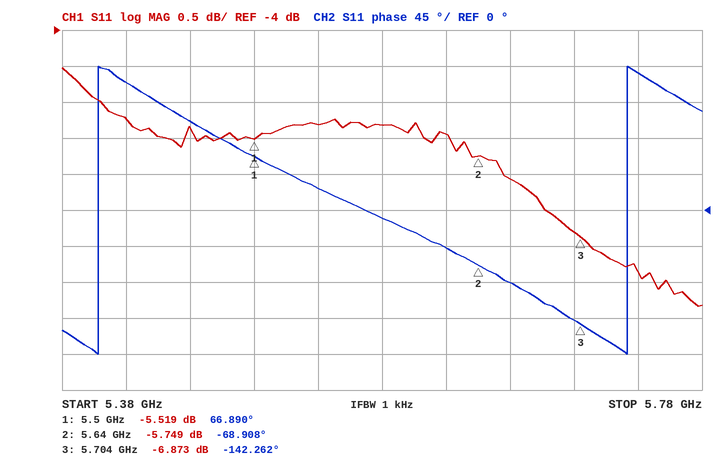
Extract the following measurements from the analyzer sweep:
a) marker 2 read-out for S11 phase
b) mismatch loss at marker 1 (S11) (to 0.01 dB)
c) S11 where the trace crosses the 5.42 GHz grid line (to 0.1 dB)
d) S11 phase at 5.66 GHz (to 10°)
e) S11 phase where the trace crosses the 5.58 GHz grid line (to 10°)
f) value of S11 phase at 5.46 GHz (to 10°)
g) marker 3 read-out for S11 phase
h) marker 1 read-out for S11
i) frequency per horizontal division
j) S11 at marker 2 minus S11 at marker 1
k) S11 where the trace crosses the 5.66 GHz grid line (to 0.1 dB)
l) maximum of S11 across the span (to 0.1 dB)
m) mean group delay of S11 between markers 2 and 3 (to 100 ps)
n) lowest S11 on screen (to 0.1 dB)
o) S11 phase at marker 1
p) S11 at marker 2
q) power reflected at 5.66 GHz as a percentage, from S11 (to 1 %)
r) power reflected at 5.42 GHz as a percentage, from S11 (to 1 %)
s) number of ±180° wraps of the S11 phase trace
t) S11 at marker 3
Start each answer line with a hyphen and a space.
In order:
- -68.908°
- 1.43 dB
- -5.2 dB
- -90°
- -10°
- 110°
- -142.262°
- -5.519 dB
- 40 MHz
- -0.230 dB
- -6.1 dB
- -4.5 dB
- 3.2 ns
- -7.8 dB
- 66.890°
- -5.749 dB
- 25 %
- 30 %
- 2
- -6.873 dB
